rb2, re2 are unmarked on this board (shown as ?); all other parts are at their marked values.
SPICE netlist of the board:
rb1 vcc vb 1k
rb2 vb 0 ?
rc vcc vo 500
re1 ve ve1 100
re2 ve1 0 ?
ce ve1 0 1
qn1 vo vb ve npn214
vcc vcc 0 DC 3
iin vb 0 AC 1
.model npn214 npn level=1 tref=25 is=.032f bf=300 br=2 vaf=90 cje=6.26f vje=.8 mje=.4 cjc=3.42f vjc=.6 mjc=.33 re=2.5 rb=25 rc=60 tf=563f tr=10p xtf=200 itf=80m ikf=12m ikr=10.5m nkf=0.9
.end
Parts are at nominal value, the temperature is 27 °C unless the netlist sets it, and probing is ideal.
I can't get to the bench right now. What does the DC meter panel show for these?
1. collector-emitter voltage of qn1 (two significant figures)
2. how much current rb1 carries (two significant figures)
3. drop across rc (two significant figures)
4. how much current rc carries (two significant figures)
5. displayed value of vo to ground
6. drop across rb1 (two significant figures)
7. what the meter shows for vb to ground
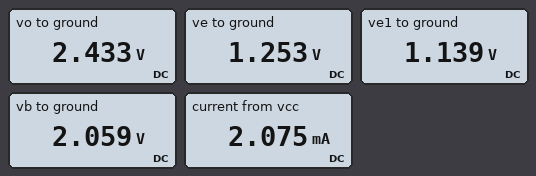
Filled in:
1.2 V
940 µA
570 mV
1.1 mA
2.433 V
940 mV
2.059 V
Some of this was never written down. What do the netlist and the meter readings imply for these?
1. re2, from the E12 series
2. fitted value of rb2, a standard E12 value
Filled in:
1 kΩ
2.2 kΩ
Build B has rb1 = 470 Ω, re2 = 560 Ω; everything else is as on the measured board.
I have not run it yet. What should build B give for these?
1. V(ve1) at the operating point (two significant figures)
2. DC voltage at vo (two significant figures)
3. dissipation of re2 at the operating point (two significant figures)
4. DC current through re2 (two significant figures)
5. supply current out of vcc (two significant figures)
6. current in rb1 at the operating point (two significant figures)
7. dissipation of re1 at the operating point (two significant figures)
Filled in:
1.4 V
1.8 V
3.3 mW
2.4 mA
3.5 mA
1.2 mA
590 µW
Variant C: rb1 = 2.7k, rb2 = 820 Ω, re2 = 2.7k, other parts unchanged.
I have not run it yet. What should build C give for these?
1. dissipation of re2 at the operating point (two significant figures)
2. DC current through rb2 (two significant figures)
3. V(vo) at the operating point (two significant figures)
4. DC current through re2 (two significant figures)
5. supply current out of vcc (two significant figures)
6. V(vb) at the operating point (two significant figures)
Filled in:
220 nW
850 µA
3.0 V
9.1 µA
860 µA
700 mV
